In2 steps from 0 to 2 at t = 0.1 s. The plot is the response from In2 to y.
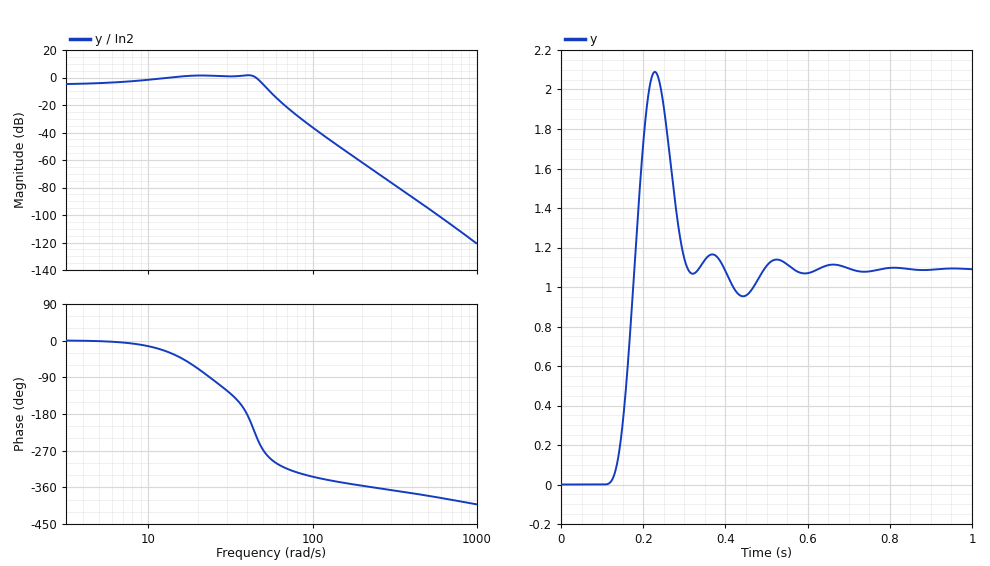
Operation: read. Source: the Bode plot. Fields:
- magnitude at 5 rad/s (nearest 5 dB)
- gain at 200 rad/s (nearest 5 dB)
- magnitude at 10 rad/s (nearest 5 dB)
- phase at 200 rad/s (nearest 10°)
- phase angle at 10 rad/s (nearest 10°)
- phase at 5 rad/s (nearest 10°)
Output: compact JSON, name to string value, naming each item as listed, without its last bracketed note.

{"magnitude at 5 rad/s": "-5 dB", "gain at 200 rad/s": "-60 dB", "magnitude at 10 rad/s": "0 dB", "phase at 200 rad/s": "-360°", "phase angle at 10 rad/s": "-10°", "phase at 5 rad/s": "0°"}
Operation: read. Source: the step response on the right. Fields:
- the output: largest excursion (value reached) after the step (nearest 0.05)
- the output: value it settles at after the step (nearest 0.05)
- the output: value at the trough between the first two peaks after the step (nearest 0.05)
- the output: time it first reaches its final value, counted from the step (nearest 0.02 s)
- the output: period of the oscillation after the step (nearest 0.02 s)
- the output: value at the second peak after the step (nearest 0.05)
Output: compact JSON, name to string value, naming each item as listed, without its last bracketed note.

{"the output: largest excursion (value reached) after the step": "2.10", "the output: value it settles at after the step": "1.10", "the output: value at the trough between the first two peaks after the step": "1.05", "the output: time it first reaches its final value, counted from the step": "0.08 s", "the output: period of the oscillation after the step": "0.14 s", "the output: value at the second peak after the step": "1.15"}
